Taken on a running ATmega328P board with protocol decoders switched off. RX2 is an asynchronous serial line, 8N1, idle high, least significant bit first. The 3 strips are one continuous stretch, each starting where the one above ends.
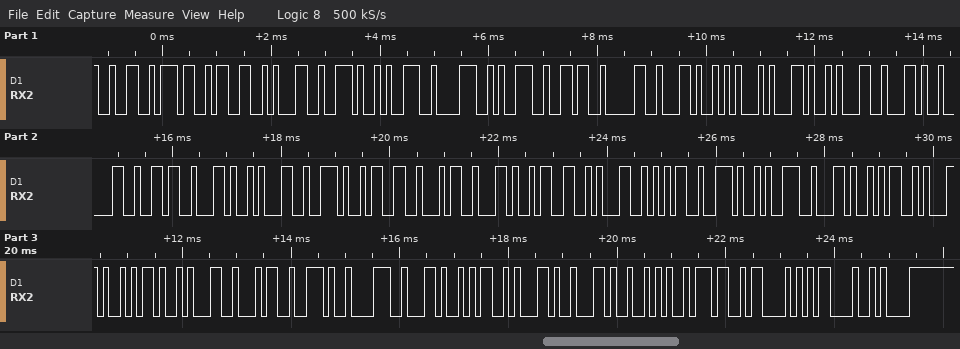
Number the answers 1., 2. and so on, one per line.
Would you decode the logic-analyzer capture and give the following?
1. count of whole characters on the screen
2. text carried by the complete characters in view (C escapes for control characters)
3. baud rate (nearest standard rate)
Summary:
1. 45
2. "2731.98960,E,1,06,1.34,315.9,M,-14.8,M,,*7C\r\n"
3. 9600 baud
